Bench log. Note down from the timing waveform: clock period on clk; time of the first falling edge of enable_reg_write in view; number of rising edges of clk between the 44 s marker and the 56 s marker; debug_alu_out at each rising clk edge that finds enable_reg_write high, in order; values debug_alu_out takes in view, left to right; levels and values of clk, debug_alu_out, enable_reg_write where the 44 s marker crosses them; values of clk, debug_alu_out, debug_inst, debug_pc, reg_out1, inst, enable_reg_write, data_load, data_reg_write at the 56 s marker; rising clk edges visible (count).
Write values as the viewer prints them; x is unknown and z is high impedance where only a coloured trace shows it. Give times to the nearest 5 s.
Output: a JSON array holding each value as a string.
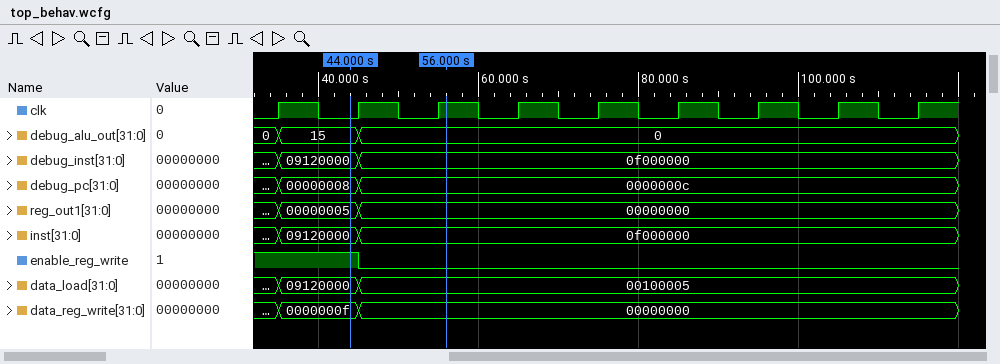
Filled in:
["10 s", "45 s", "2", "0, 15", "0, 15, 0", "clk=0, debug_alu_out=15, enable_reg_write=1", "clk=1, debug_alu_out=0, debug_inst=0f000000, debug_pc=0000000c, reg_out1=00000000, inst=0f000000, enable_reg_write=0, data_load=00100005, data_reg_write=00000000", "9"]
